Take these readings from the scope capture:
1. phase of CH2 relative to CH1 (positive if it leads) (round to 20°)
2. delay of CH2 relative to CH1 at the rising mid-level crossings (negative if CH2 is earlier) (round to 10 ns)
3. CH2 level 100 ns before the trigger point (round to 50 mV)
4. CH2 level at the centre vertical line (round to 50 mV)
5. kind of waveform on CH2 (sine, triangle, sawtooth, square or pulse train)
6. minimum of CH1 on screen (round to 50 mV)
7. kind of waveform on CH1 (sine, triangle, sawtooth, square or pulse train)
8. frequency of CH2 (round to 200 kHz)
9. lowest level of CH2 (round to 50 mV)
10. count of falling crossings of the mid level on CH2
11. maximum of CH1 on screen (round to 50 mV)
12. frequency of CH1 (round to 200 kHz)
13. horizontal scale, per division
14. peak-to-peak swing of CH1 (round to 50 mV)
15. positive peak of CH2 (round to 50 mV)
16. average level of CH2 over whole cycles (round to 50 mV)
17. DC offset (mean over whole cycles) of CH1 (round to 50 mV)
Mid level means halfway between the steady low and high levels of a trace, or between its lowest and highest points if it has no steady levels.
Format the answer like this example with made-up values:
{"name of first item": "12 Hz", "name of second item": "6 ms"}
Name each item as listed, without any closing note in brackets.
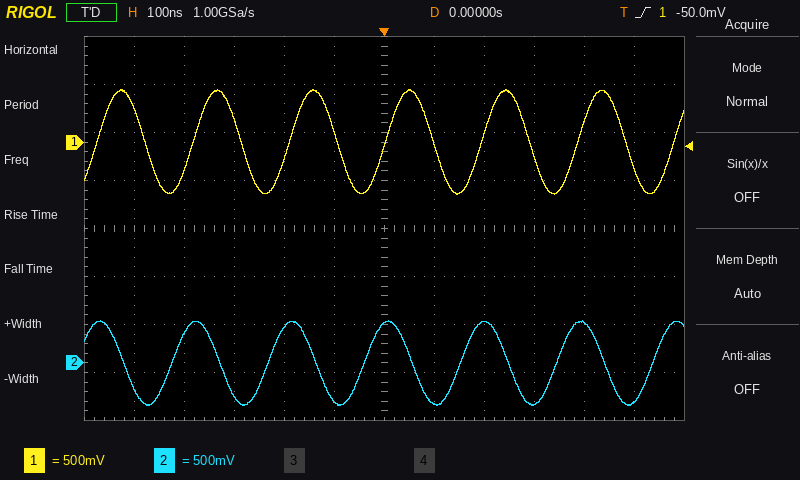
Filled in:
{"phase of CH2 relative to CH1 (positive if it leads)": "+80°", "delay of CH2 relative to CH1 at the rising mid-level crossings (negative if CH2 is earlier)": "-40 ns", "CH2 level 100 ns before the trigger point": "-400 mV", "CH2 level at the centre vertical line": "400 mV", "kind of waveform on CH2": "sine", "minimum of CH1 on screen": "-550 mV", "kind of waveform on CH1": "sine", "frequency of CH2": "5.2 MHz", "lowest level of CH2": "-450 mV", "count of falling crossings of the mid level on CH2": "6", "maximum of CH1 on screen": "550 mV", "frequency of CH1": "5.2 MHz", "horizontal scale, per division": "100 ns", "peak-to-peak swing of CH1": "1.10 V", "positive peak of CH2": "450 mV", "average level of CH2 over whole cycles": "0 mV", "DC offset (mean over whole cycles) of CH1": "0 mV"}
